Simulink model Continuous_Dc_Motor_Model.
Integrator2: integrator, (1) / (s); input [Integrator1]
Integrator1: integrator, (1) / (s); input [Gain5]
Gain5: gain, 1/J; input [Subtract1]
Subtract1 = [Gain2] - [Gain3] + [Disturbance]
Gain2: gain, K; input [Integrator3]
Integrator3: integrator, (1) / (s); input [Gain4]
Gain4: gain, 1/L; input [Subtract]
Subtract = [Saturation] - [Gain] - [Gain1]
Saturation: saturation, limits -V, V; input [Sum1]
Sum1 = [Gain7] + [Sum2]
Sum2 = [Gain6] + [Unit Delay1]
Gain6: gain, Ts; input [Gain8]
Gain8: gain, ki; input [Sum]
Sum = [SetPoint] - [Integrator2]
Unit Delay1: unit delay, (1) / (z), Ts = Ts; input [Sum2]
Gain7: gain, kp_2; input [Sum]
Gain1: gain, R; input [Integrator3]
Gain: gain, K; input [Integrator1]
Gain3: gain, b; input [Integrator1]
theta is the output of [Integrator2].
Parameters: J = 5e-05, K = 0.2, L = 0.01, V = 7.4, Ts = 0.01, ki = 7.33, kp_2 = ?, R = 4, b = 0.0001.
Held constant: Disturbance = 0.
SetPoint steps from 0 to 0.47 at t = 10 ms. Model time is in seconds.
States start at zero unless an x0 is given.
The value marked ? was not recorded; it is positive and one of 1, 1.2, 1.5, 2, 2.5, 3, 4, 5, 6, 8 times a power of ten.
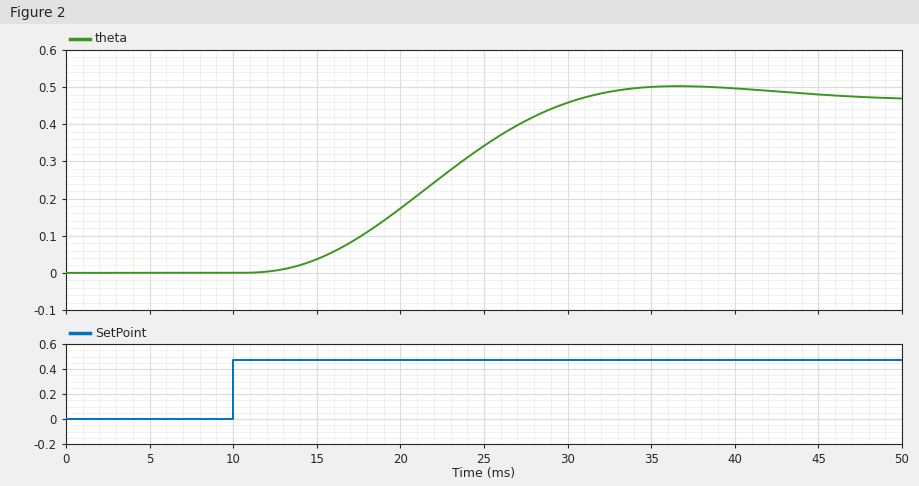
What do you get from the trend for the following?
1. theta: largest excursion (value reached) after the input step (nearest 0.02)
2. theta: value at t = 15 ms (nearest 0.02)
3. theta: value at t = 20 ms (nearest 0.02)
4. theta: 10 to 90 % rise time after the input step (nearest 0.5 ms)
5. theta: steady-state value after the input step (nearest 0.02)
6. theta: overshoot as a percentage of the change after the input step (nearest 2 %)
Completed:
0.50
0.04
0.18
12.5 ms
0.48
6 %
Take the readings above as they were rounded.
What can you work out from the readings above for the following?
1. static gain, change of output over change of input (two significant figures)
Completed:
1.0
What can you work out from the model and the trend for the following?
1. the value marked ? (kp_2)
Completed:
20
